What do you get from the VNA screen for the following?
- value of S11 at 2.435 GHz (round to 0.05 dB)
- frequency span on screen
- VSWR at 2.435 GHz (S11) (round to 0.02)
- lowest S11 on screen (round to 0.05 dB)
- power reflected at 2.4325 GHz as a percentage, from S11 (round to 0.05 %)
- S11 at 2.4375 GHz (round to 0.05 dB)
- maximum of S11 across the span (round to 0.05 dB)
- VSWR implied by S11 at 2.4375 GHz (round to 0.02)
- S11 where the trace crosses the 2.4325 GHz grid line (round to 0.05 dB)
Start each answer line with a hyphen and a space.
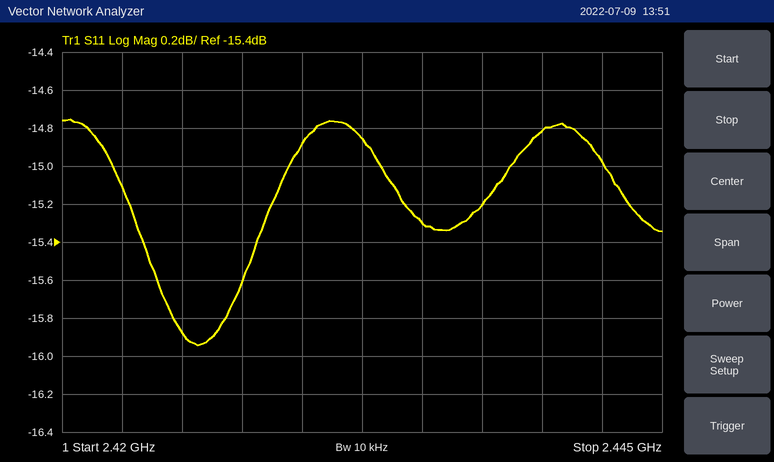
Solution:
- -15.30 dB
- 25 MHz
- 1.42
- -15.95 dB
- 3.25 %
- -15.20 dB
- -14.75 dB
- 1.42
- -14.85 dB
